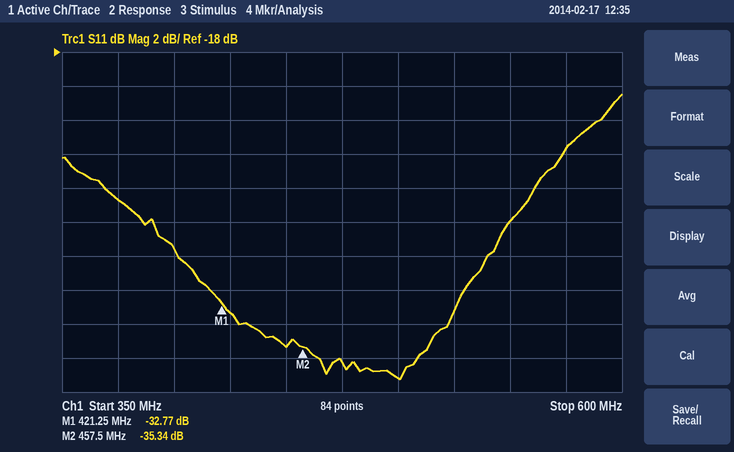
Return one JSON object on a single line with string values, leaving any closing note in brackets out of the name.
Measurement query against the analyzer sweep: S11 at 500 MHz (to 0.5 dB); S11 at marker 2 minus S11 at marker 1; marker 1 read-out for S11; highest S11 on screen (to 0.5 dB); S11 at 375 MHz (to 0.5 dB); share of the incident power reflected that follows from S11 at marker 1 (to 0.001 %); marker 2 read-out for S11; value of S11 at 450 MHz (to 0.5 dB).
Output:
{"S11 at 500 MHz": "-37.0 dB", "S11 at marker 2 minus S11 at marker 1": "-2.57 dB", "marker 1 read-out for S11": "-32.77 dB", "highest S11 on screen": "-20.5 dB", "S11 at 375 MHz": "-26.5 dB", "share of the incident power reflected that follows from S11 at marker 1": "0.053 %", "marker 2 read-out for S11": "-35.34 dB", "value of S11 at 450 MHz": "-35.5 dB"}
